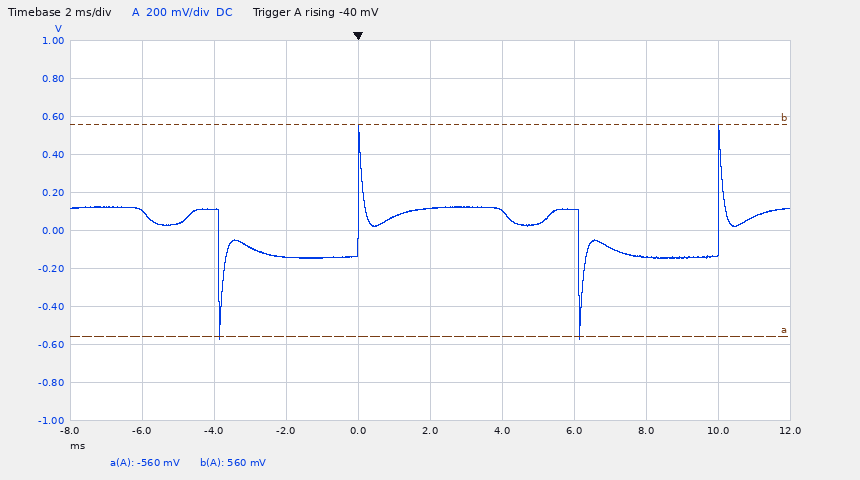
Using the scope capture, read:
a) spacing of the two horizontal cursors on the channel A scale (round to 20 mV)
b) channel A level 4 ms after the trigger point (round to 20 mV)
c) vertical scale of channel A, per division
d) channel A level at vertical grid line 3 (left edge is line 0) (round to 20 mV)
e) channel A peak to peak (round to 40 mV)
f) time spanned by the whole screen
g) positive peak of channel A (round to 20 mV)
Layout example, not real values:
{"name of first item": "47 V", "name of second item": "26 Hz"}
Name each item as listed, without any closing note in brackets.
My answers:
{"spacing of the two horizontal cursors on the channel A scale": "1.12 V", "channel A level 4 ms after the trigger point": "100 mV", "vertical scale of channel A, per division": "200 mV", "channel A level at vertical grid line 3 (left edge is line 0)": "-140 mV", "channel A peak to peak": "1.12 V", "time spanned by the whole screen": "20 ms", "positive peak of channel A": "560 mV"}
